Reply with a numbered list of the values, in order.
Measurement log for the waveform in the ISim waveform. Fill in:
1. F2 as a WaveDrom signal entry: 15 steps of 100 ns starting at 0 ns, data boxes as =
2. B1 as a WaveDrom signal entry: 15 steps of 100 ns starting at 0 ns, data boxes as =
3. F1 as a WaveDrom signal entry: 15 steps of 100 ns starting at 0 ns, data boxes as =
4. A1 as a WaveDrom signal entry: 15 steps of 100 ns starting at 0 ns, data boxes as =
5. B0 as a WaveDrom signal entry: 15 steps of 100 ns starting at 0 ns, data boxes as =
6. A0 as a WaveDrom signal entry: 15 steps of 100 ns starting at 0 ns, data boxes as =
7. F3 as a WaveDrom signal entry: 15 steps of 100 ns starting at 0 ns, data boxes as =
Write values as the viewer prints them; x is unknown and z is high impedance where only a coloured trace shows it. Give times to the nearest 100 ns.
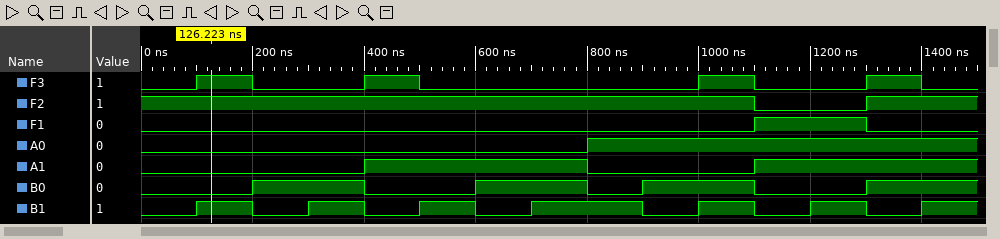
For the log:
1. {name: 'F2', wave: '1..........0.1.'}
2. {name: 'B1', wave: '01010101.010101'}
3. {name: 'F1', wave: '0..........1.0.'}
4. {name: 'A1', wave: '0...1...0..1...'}
5. {name: 'B0', wave: '0.1.0.1.01.0.1.'}
6. {name: 'A0', wave: '0.......1......'}
7. {name: 'F3', wave: '010.10....10.10'}
